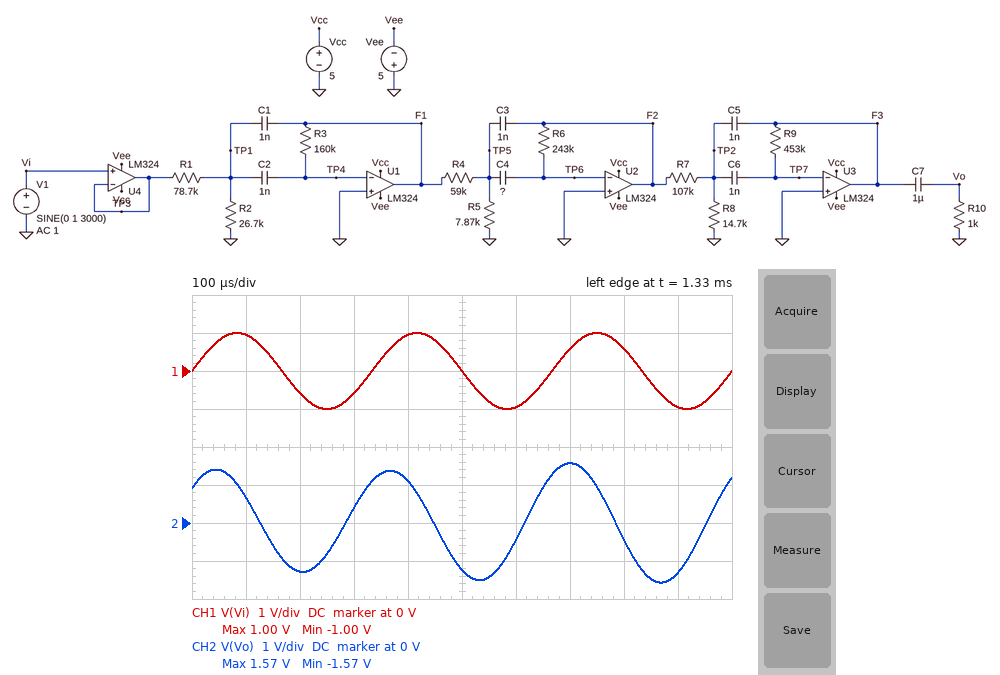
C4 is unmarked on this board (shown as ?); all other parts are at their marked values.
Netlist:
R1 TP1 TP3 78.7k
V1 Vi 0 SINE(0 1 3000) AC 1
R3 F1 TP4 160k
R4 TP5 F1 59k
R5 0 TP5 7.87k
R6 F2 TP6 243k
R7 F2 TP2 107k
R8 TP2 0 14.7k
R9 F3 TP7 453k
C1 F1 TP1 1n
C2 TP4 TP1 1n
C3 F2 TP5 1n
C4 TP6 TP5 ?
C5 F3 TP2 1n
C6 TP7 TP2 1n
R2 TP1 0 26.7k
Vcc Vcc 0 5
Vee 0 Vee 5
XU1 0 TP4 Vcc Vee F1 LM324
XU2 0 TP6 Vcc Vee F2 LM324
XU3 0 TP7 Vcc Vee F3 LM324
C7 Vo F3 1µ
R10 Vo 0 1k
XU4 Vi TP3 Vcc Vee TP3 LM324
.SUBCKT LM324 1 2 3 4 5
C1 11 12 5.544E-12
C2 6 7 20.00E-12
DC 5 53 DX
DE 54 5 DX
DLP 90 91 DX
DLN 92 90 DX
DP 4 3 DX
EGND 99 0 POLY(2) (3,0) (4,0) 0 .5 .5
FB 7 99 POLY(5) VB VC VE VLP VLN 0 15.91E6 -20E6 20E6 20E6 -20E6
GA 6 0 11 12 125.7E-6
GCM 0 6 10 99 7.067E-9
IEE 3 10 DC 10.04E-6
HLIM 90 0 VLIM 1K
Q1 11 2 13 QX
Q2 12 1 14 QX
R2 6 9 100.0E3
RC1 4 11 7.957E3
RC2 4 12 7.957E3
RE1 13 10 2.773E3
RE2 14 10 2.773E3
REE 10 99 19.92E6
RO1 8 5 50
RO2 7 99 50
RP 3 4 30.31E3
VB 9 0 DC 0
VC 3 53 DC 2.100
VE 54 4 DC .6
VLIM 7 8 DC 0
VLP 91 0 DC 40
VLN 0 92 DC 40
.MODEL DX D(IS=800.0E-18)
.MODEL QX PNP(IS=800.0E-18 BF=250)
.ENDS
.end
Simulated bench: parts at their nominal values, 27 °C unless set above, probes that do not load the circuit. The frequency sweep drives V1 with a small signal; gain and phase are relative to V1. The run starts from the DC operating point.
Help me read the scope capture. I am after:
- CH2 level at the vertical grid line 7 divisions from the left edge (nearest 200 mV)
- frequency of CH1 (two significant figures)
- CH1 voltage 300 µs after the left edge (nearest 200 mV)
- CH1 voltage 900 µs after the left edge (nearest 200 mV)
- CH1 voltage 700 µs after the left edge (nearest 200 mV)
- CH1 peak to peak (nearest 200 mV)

1.6 V
3.0 kHz
-600 mV
-1.0 V
600 mV
2.0 V
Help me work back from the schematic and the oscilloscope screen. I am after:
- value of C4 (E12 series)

2.7 nF
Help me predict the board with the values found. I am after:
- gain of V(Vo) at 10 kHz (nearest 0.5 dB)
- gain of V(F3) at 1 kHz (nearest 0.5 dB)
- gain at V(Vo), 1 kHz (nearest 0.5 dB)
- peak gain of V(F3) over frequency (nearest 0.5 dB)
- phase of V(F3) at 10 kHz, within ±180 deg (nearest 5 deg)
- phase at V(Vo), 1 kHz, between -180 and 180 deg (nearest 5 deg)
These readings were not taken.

-41.0 dB
-23.0 dB
-23.0 dB
13.5 dB
-70 deg
60 deg
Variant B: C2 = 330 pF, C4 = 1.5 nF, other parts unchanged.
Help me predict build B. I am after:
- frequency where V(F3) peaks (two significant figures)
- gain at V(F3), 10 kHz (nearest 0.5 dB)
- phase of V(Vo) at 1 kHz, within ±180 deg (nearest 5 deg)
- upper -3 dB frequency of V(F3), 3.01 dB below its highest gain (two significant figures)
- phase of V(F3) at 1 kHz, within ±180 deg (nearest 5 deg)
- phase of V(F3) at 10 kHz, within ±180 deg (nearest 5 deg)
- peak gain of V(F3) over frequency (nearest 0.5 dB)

3.0 kHz
-39.5 dB
70 deg
3.6 kHz
60 deg
-55 deg
-4.0 dB
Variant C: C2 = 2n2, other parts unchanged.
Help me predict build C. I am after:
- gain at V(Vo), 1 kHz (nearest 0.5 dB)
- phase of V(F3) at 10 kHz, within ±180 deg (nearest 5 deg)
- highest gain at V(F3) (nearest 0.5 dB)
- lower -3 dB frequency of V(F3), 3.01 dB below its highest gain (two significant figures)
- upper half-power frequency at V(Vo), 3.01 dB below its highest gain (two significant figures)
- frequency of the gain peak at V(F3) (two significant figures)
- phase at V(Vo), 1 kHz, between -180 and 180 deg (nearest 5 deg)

-15.5 dB
-75 deg
17.5 dB
1.9 kHz
2.4 kHz
2.1 kHz
45 deg
